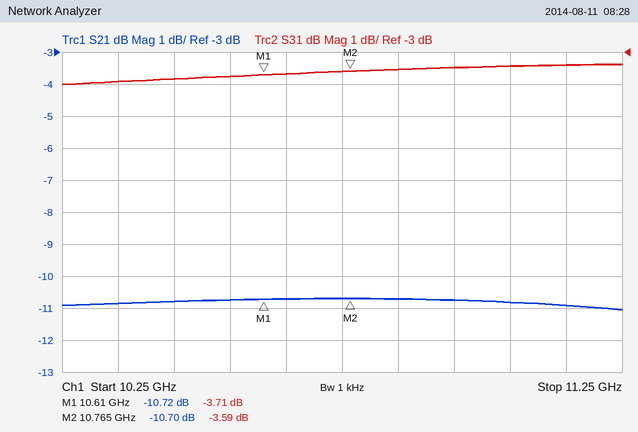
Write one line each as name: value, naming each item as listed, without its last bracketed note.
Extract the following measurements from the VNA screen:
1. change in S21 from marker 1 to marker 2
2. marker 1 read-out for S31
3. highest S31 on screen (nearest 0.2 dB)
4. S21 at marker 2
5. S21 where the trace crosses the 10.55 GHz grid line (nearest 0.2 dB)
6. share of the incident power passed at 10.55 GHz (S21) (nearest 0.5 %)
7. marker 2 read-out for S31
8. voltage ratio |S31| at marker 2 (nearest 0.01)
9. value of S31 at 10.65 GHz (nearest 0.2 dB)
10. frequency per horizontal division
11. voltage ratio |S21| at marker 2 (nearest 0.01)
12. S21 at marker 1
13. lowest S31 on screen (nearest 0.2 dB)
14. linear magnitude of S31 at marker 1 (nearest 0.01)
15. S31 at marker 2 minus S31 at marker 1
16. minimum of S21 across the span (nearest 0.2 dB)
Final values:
change in S21 from marker 1 to marker 2: 0.02 dB
marker 1 read-out for S31: -3.71 dB
highest S31 on screen: -3.4 dB
S21 at marker 2: -10.70 dB
S21 where the trace crosses the 10.55 GHz grid line: -10.8 dB
share of the incident power passed at 10.55 GHz (S21): 8.5 %
marker 2 read-out for S31: -3.59 dB
voltage ratio |S31| at marker 2: 0.66
value of S31 at 10.65 GHz: -3.6 dB
frequency per horizontal division: 100 MHz
voltage ratio |S21| at marker 2: 0.29
S21 at marker 1: -10.72 dB
lowest S31 on screen: -4.0 dB
linear magnitude of S31 at marker 1: 0.65
S31 at marker 2 minus S31 at marker 1: 0.12 dB
minimum of S21 across the span: -11.0 dB
